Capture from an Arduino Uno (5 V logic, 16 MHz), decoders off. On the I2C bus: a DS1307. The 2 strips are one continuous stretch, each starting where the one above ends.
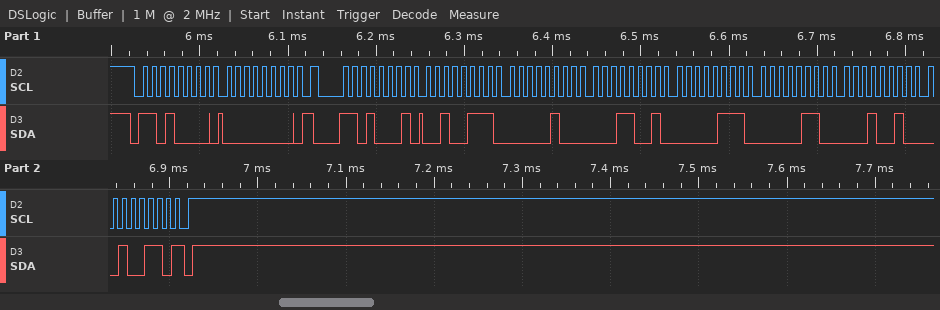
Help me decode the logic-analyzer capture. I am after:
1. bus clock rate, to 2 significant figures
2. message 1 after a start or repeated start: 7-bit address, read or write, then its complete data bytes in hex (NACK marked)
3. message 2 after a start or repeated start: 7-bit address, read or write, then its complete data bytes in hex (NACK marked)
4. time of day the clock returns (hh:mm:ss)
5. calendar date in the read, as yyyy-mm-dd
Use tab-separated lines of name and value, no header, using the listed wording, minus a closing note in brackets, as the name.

bus clock rate, to 2 significant figures	100 kHz
message 1 after a start or repeated start: 7-bit address, read or write, then its complete data bytes in hex	0x68 write: 00
message 2 after a start or repeated start: 7-bit address, read or write, then its complete data bytes in hex	0x68 read: 27 04 19 07 06 12 26 NACK
time of day the clock returns	19:04:27
calendar date in the read, as yyyy-mm-dd	2026-12-06
